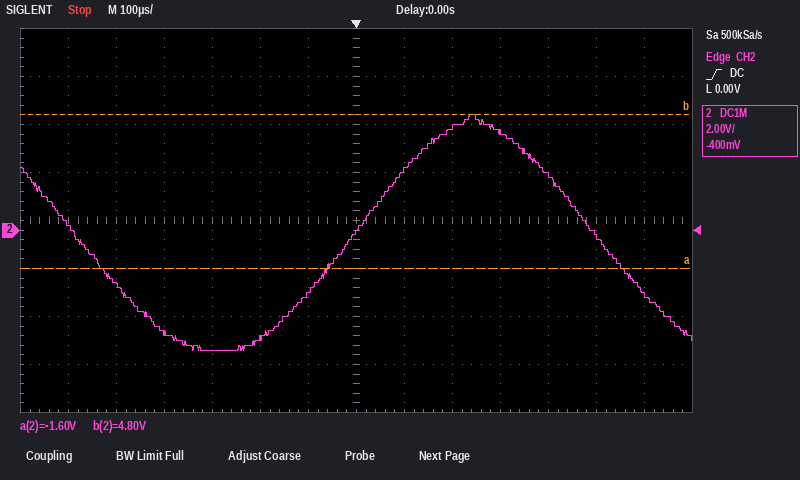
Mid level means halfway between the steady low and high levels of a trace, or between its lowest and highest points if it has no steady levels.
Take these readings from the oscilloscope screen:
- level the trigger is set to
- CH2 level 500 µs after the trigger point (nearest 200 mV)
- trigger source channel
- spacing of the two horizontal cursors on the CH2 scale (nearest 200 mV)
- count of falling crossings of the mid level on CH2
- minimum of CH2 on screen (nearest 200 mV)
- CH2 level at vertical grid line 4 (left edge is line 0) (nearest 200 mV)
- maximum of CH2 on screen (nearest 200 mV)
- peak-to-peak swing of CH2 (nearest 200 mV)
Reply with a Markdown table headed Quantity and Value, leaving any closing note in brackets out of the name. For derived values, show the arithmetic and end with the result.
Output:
| Quantity | Value |
|---|---|
| level the trigger is set to | 0.00 V |
| CH2 level 500 µs after the trigger point | -200 mV |
| trigger source channel | CH2 |
| spacing of the two horizontal cursors on the CH2 scale | 6.4 V |
| count of falling crossings of the mid level on CH2 | 2 |
| minimum of CH2 on screen | -5.0 V |
| CH2 level at vertical grid line 4 (left edge is line 0) | -5.0 V |
| maximum of CH2 on screen | 4.8 V |
| peak-to-peak swing of CH2 | 4.8 V − (-5.0 V) = 9.8 V |
